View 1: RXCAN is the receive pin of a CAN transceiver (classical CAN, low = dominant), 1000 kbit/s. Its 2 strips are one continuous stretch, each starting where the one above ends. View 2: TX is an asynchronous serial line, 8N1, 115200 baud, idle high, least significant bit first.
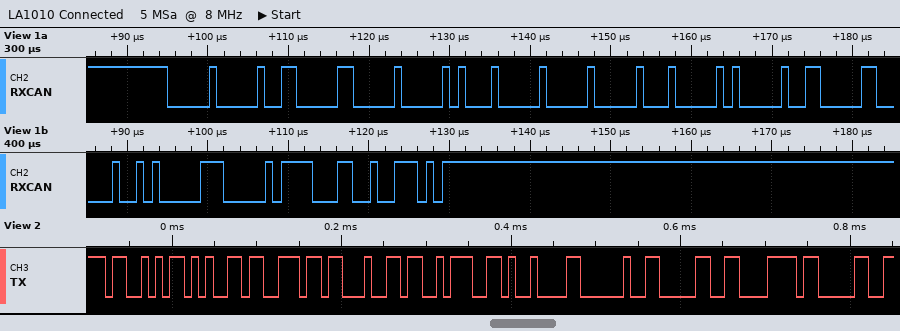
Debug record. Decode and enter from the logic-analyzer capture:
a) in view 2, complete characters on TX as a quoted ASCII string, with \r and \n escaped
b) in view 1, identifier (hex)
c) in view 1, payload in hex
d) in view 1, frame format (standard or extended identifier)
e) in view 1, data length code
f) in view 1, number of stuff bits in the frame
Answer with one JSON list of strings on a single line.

["\"Send:\\t 0x0\"", "0x00001001", "00 01 02 03 04 05 06 07", "extended", "8", "14"]
